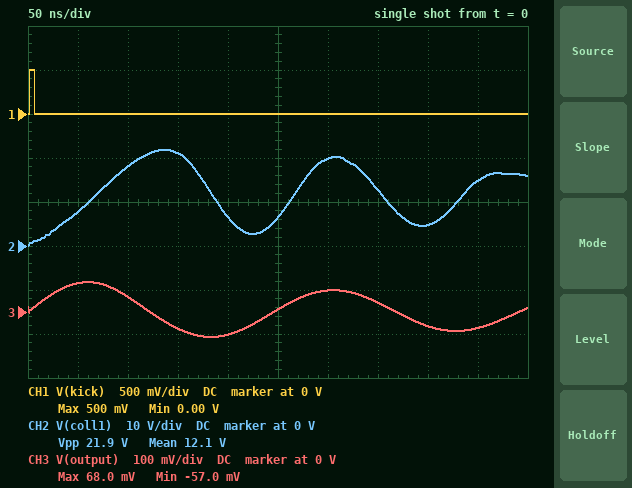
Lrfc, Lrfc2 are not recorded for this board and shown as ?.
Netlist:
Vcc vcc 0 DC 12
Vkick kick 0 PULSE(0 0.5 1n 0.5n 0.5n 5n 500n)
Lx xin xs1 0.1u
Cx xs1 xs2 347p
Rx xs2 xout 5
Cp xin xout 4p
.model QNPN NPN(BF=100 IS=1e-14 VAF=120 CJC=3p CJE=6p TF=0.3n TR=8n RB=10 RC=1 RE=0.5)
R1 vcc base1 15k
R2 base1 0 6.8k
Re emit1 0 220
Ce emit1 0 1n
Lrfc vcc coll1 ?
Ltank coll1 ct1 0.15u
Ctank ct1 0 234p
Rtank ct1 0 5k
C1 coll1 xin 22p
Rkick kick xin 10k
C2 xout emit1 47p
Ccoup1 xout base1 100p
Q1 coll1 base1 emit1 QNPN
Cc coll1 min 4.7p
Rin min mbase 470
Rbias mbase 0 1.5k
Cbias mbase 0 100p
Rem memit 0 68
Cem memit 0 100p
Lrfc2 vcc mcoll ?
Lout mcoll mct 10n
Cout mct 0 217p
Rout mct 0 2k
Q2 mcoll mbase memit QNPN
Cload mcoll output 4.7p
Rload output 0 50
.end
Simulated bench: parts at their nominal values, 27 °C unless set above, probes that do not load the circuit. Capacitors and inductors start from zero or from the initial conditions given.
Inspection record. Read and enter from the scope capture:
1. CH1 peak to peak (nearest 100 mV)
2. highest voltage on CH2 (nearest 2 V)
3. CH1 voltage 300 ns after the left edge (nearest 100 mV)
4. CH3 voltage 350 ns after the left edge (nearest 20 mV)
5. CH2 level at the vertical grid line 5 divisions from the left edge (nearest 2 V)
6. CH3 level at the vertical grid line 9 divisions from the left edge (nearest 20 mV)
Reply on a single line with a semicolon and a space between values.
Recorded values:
500 mV; 22 V; 0 V; 20 mV; 6 V; -40 mV
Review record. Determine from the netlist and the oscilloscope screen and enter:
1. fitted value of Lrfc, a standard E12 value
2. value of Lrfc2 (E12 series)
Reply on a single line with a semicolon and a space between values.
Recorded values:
2.7 µH; 6.8 µH
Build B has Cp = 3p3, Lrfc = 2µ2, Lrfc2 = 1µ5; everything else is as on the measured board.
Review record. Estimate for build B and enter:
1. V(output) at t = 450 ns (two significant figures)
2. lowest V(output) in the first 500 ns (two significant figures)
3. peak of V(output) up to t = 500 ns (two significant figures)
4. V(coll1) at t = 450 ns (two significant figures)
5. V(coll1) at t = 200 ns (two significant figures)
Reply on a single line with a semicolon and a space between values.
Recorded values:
-53 mV; -140 mV; 150 mV; 16 V; 3.4 V
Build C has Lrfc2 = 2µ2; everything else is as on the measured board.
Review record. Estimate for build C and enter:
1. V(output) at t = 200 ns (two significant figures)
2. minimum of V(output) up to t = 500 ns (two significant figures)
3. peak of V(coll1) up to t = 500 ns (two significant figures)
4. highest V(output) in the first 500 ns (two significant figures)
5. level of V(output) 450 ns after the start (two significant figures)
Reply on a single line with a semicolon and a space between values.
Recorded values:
41 mV; -110 mV; 22 V; 120 mV; 75 mV
